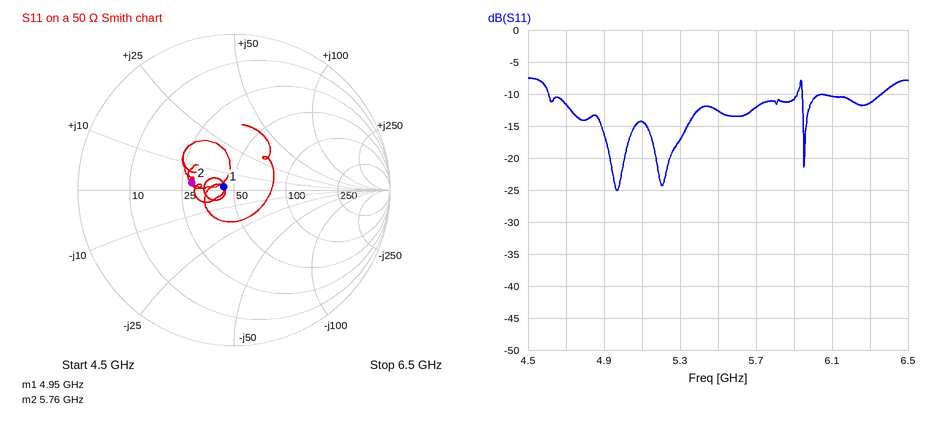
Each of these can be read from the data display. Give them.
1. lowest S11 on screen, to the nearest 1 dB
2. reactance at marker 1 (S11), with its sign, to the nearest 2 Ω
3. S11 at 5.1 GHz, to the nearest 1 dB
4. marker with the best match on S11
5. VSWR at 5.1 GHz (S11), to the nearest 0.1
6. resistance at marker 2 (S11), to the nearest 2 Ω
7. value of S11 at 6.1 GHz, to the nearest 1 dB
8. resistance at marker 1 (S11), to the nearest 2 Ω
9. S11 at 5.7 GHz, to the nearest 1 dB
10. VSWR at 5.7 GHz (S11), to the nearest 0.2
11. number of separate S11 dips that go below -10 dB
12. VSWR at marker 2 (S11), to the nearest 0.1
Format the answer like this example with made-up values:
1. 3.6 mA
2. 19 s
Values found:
1. -25 dB
2. +2 Ω
3. -14 dB
4. marker 1
5. 1.5
6. 28 Ω
7. -10 dB
8. 44 Ω
9. -12 dB
10. 1.6
11. 3
12. 1.8
